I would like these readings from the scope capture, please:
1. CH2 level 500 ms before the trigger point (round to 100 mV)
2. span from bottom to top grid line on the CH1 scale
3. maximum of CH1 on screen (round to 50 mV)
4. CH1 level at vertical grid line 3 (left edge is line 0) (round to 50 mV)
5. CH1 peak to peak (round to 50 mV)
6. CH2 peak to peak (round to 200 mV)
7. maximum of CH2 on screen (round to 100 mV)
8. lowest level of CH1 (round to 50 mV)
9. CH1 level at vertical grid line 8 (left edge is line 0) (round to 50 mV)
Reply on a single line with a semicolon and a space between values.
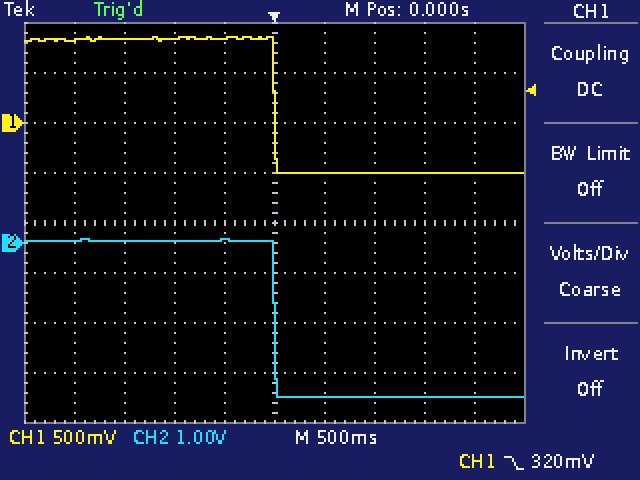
100 mV; 4 V; 850 mV; 850 mV; 1.35 V; 3.2 V; 100 mV; -500 mV; -500 mV
